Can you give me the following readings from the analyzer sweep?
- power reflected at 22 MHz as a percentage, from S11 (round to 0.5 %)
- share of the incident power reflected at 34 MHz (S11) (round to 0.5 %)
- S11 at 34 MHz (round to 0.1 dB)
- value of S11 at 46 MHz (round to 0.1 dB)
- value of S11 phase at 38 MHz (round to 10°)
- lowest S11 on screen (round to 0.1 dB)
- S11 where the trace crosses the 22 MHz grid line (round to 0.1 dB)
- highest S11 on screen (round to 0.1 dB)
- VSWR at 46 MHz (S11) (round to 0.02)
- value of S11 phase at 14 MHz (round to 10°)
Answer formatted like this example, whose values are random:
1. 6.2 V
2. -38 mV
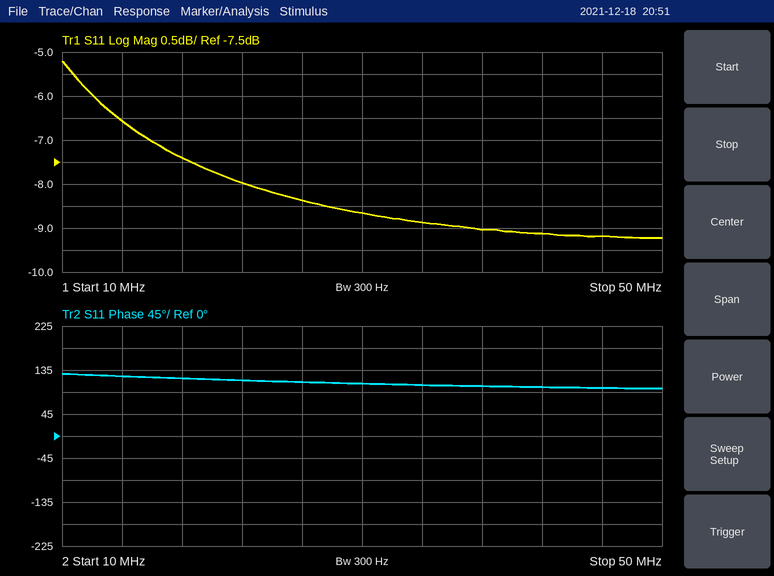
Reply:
1. 16.0 %
2. 13.0 %
3. -8.9 dB
4. -9.2 dB
5. 100°
6. -9.2 dB
7. -8.0 dB
8. -5.2 dB
9. 2.06
10. 120°
